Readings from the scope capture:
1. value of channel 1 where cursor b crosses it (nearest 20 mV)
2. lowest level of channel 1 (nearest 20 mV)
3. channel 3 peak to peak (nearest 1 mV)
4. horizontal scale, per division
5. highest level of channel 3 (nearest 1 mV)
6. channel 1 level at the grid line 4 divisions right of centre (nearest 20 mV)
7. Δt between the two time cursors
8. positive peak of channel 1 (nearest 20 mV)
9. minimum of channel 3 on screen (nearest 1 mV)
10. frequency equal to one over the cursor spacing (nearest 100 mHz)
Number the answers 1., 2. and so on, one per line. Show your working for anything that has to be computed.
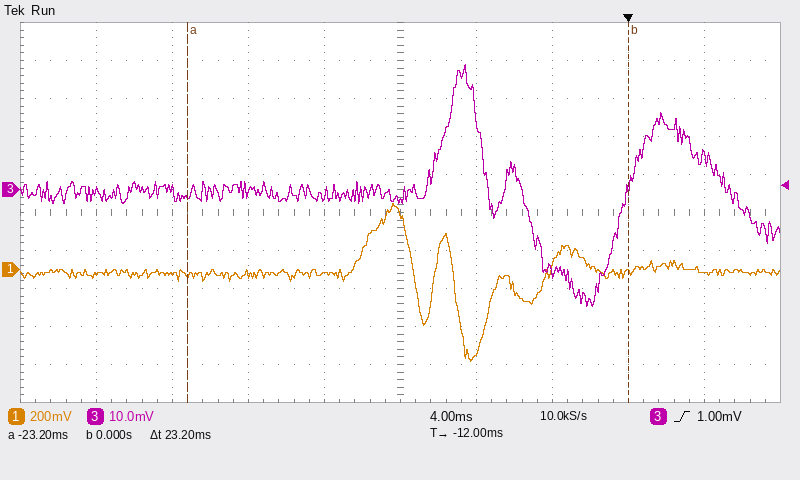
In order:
1. -20 mV
2. -480 mV
3. 33 mV − (-31 mV) = 64 mV
4. 4 ms
5. 33 mV
6. -20 mV
7. 23.2 ms
8. 340 mV
9. -31 mV
10. 1 / 23.2 ms ≈ 43.1 Hz
